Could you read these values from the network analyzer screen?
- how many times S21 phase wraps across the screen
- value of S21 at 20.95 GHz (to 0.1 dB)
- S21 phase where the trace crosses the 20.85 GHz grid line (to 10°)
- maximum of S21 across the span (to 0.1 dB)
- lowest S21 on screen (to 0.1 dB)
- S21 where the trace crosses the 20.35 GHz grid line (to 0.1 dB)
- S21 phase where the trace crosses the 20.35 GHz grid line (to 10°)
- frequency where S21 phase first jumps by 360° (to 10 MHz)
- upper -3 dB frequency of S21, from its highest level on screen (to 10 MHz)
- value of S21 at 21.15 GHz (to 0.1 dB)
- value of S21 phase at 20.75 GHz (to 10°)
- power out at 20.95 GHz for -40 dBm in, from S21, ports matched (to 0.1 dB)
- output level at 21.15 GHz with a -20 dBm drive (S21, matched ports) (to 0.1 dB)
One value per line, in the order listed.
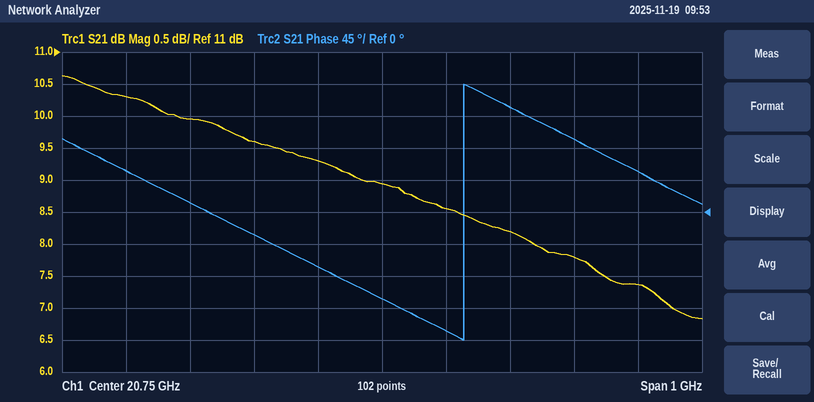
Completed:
1
8.2 dB
-170°
10.6 dB
6.8 dB
10.3 dB
60°
20.88 GHz
21.08 GHz
7.4 dB
-120°
-31.8 dBm
-12.6 dBm
